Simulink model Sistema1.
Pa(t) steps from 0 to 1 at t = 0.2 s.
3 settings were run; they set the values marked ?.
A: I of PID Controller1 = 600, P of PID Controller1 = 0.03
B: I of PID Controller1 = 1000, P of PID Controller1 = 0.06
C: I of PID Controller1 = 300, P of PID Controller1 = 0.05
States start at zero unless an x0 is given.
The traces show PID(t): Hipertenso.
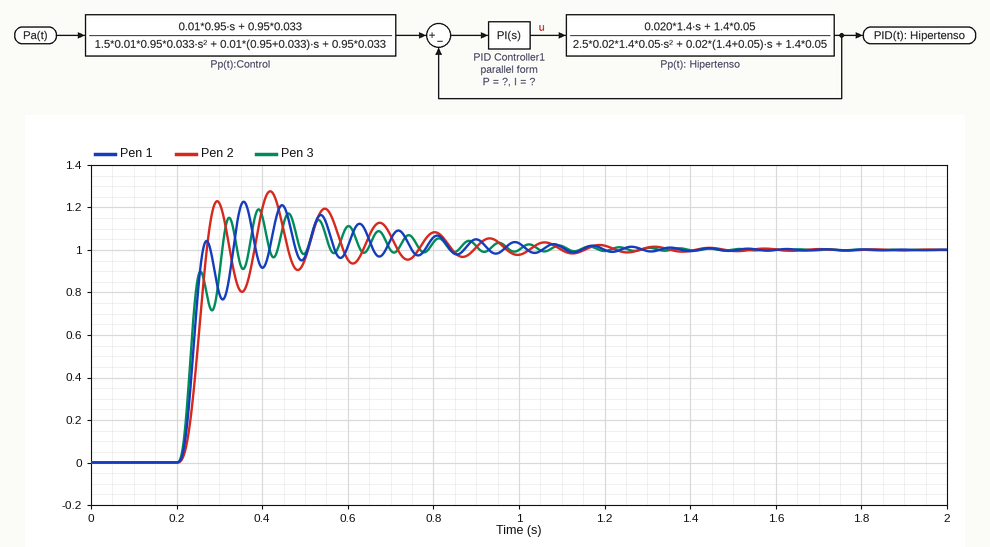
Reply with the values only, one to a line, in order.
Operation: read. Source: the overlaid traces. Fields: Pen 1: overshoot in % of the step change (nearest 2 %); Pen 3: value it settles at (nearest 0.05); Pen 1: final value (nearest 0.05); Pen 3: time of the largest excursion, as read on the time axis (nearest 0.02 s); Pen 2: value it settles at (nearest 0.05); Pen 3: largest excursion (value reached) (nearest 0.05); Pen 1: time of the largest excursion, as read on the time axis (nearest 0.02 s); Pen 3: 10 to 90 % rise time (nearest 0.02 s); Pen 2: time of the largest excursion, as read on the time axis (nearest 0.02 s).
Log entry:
22 %
1.00
1.00
0.40 s
1.00
1.20
0.36 s
0.08 s
0.42 s
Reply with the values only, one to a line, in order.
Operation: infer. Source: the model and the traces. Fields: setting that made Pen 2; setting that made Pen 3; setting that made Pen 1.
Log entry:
C
B
A
